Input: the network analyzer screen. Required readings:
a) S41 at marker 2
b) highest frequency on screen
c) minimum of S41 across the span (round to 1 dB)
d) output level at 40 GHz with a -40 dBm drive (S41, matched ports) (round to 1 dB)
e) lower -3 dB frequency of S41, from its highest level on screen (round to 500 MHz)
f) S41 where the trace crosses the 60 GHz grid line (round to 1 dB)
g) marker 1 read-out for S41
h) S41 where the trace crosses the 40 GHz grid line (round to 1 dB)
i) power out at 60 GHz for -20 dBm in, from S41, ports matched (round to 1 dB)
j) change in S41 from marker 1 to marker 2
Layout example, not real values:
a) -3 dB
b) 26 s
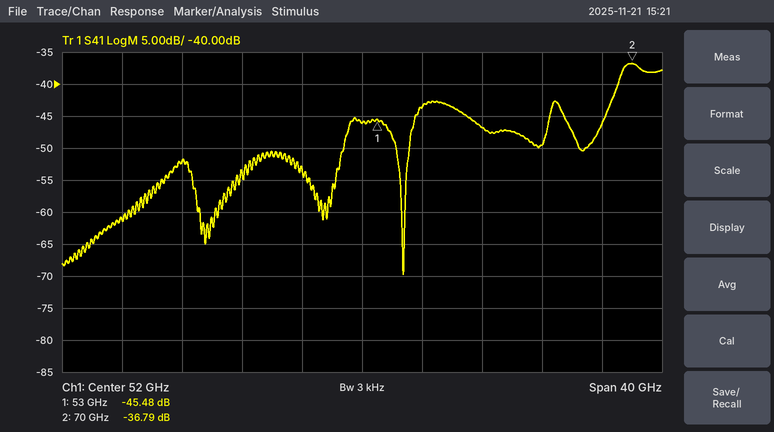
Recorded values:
a) -36.79 dB
b) 72 GHz
c) -70 dB
d) -92 dBm
e) 69.0 GHz
f) -47 dB
g) -45.48 dB
h) -52 dB
i) -67 dBm
j) 8.69 dB
